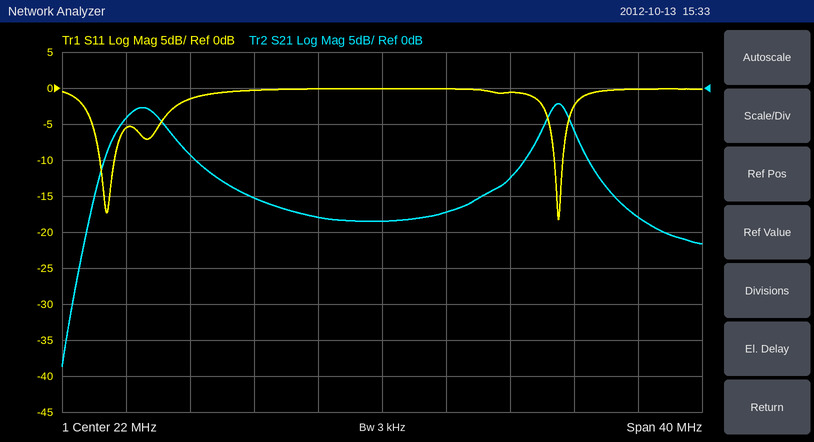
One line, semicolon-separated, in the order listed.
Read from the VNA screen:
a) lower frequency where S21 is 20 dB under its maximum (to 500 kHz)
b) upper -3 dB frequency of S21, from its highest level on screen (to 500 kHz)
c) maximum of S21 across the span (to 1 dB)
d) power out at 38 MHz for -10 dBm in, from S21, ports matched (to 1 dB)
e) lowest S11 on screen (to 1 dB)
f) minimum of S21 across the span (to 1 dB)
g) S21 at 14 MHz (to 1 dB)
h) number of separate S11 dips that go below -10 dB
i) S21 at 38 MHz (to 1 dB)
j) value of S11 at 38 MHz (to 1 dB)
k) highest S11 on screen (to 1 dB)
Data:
3.5 MHz; 34.0 MHz; -2 dB; -28 dBm; -18 dB; -39 dB; -15 dB; 2; -18 dB; 0 dB; 0 dB
